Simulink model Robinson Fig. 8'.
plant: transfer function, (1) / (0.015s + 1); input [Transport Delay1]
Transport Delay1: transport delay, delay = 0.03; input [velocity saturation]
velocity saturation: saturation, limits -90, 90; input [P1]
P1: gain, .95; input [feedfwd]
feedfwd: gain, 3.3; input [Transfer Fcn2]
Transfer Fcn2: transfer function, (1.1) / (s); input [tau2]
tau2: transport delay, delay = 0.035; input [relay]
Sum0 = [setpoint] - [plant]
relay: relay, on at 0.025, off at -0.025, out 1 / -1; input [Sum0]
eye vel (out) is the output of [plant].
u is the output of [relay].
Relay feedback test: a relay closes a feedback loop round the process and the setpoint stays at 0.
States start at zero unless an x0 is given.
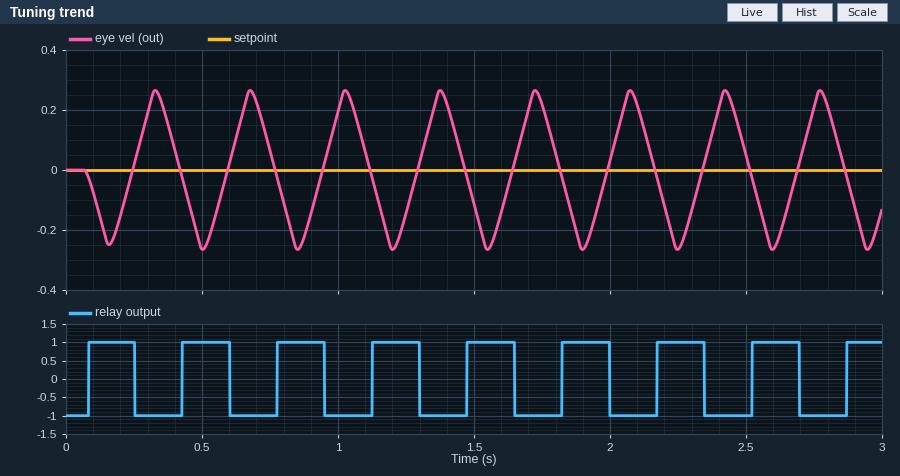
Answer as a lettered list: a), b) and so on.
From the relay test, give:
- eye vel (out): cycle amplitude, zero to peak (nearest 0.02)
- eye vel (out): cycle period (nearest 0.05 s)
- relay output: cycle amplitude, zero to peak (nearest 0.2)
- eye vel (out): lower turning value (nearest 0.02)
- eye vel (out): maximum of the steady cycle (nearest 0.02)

a) 0.26
b) 0.35 s
c) 1.0
d) -0.26
e) 0.26
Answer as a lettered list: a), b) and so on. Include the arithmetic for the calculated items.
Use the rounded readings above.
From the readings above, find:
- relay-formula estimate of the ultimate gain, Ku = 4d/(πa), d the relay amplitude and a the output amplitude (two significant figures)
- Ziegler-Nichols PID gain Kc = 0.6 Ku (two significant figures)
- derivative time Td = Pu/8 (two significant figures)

a) 4 × 1 / (π × 0.26) = 4.9
b) 0.6 × 4.9 = 2.9
c) 0.35 / 8 = 0.044 s
